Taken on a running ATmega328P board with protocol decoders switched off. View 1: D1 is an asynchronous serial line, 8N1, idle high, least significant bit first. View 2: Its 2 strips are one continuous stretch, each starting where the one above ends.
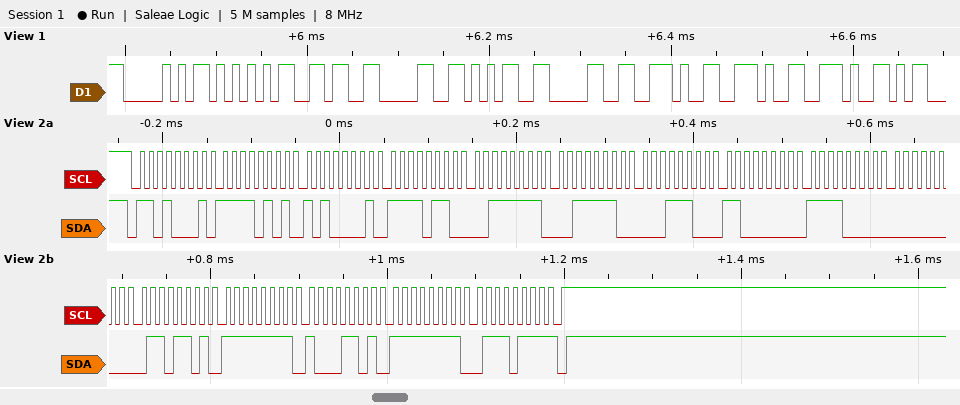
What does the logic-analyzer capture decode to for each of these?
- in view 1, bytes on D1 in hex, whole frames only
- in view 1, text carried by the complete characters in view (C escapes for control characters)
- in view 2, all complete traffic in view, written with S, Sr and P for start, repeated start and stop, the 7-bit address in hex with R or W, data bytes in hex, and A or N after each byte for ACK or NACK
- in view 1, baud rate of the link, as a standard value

50 55 36 30 35 30 2E 2E 2E
"PU6050..."
S 68R A F5 A A1 A F6 A 3F A 3E A 1C A C0 A F0 A 00 A 6D A FF A 8D A FF A 77 N P
115200 baud
